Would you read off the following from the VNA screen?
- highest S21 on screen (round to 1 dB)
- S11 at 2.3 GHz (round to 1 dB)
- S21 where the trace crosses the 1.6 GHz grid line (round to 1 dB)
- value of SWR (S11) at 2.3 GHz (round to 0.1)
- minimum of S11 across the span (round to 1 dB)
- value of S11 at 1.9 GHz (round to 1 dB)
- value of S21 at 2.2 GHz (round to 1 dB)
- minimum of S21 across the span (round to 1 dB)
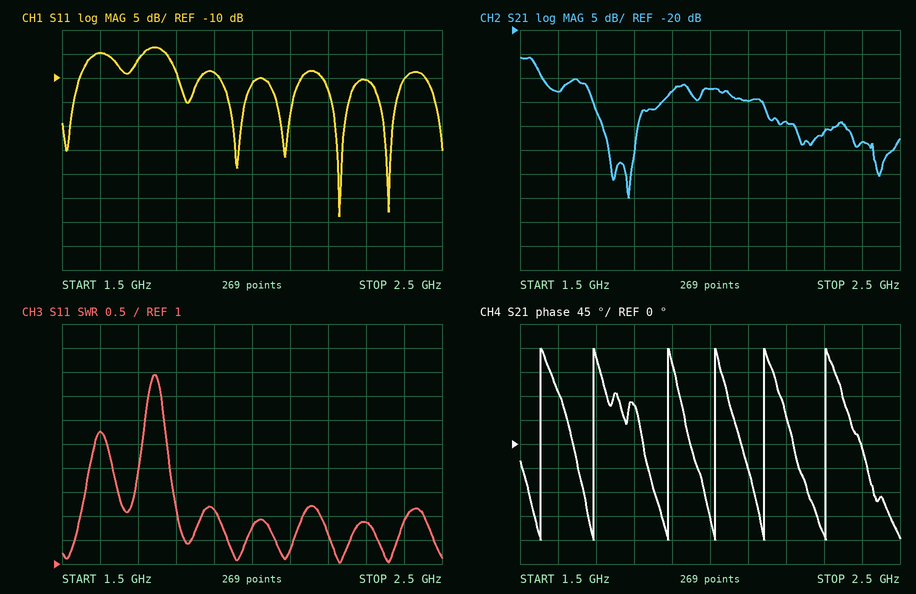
-26 dB
-10 dB
-33 dB
1.9
-39 dB
-9 dB
-39 dB
-55 dB
